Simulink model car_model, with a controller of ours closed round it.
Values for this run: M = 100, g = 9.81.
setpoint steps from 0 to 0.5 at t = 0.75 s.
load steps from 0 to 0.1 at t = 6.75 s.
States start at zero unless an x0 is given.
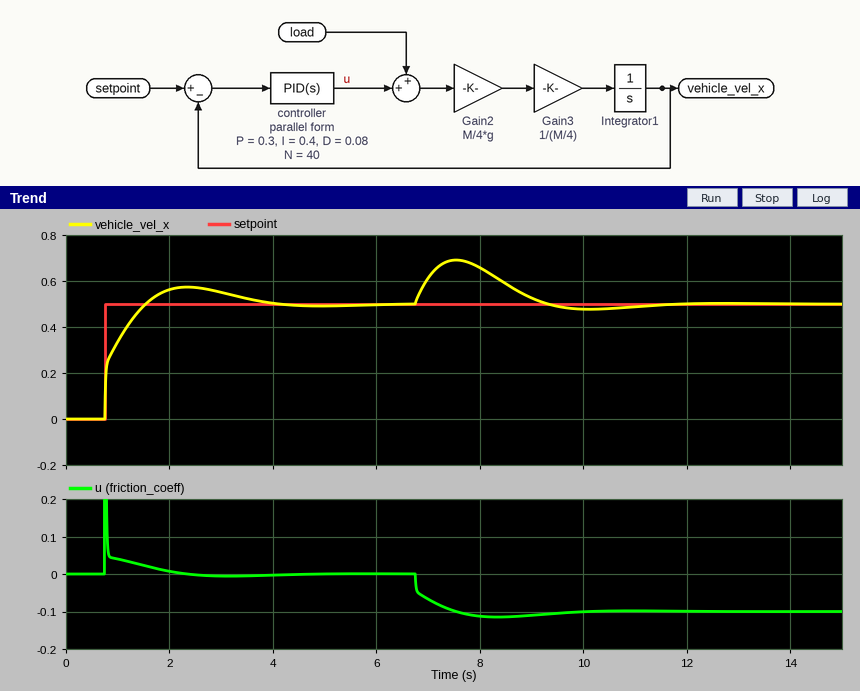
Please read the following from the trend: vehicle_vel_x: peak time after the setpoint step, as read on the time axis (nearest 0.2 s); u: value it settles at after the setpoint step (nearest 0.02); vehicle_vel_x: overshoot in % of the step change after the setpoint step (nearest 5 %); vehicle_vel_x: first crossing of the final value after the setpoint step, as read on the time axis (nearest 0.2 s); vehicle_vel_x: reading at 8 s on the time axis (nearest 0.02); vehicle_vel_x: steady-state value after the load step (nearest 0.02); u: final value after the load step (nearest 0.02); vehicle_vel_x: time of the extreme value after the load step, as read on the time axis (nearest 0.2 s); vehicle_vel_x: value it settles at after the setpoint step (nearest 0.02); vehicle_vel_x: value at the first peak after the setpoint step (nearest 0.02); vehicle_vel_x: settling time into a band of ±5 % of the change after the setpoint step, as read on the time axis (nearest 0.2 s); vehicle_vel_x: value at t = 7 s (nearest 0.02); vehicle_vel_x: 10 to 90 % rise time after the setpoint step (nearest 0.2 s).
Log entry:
2.4 s
0.00
15 %
1.6 s
0.66
0.50
-0.10
7.6 s
0.50
0.58
3.4 s
0.62
0.6 s
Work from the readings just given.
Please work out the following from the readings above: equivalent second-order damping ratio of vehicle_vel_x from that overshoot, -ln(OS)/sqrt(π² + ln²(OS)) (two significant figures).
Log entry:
0.52
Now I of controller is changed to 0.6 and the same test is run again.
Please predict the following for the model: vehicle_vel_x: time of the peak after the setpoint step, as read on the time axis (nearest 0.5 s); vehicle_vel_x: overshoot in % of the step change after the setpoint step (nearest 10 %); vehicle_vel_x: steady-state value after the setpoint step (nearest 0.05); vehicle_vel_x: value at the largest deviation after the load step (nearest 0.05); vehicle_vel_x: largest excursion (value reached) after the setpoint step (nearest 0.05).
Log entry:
2.0 s
20 %
0.50
0.65
0.60
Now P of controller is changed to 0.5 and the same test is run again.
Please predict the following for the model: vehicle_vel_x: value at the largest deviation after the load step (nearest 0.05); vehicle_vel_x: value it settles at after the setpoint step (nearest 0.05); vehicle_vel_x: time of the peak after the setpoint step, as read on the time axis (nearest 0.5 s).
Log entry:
0.65
0.50
2.0 s
